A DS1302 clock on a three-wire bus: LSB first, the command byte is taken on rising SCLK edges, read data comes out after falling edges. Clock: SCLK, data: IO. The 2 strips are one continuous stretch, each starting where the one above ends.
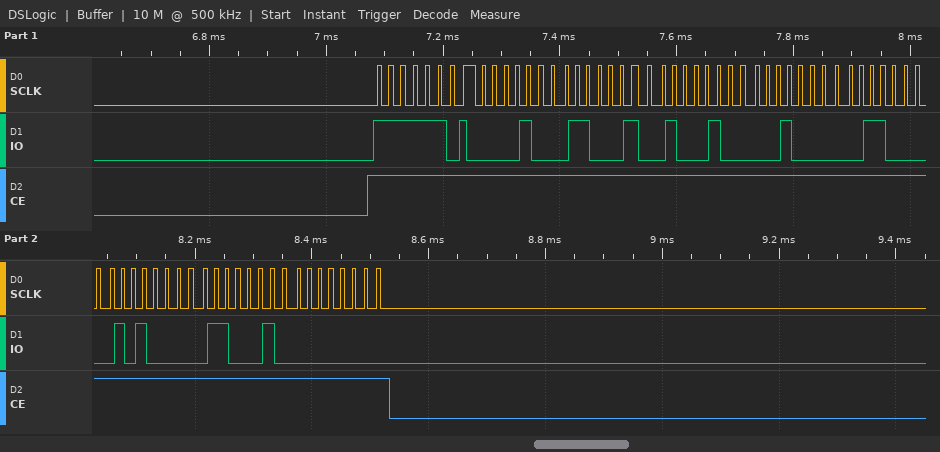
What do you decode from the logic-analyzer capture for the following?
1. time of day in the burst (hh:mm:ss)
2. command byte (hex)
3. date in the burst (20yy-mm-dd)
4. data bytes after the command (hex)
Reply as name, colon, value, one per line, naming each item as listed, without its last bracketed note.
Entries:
time of day in the burst: 11:23:10
command byte: 0xBF
date in the burst: 2023-06-04
data bytes after the command: 10 23 11 04 06 05 23 00
